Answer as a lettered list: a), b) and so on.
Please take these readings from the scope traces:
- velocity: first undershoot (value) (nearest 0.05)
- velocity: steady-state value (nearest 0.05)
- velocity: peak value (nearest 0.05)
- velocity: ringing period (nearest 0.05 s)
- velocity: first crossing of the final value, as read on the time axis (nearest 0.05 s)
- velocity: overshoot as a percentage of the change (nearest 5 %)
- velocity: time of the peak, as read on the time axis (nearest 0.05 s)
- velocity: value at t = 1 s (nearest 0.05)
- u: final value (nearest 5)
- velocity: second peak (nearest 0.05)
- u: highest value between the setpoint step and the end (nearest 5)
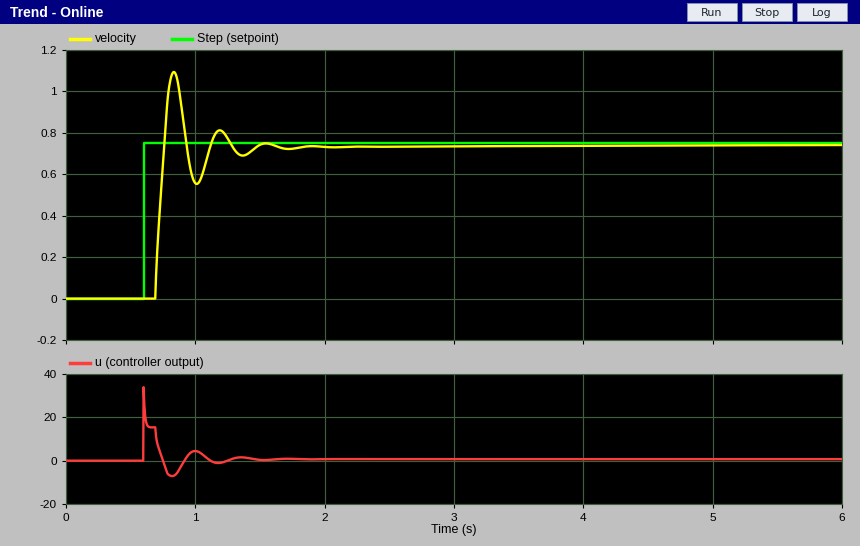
a) 0.55
b) 0.75
c) 1.10
d) 0.35 s
e) 0.75 s
f) 45 %
g) 0.85 s
h) 0.55
i) 0
j) 0.80
k) 35
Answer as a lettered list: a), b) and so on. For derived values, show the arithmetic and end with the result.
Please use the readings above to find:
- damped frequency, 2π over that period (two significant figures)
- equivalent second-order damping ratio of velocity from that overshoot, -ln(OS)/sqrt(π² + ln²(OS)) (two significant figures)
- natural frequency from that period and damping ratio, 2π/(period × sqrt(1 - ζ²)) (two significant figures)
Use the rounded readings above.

a) 2π / 0.35 = 18 rad/s
b) ln(0.45) = -0.799; 0.799 / sqrt(9.870 + 0.638) = 0.25
c) 2π / (0.35 × sqrt(1 - 0.25²)) = 19 rad/s
